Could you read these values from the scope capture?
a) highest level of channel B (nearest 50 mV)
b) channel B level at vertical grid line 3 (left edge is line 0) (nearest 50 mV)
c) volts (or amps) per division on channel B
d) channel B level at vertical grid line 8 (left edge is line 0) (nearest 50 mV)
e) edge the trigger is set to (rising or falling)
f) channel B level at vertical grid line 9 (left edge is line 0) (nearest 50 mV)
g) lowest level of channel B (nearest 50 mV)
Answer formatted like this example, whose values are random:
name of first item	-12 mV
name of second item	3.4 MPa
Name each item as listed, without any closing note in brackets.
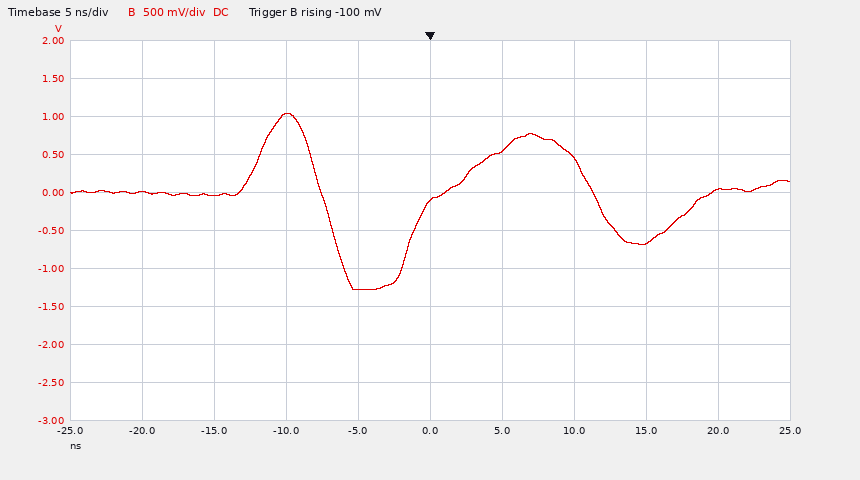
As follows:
highest level of channel B	1.05 V
channel B level at vertical grid line 3 (left edge is line 0)	1.05 V
volts (or amps) per division on channel B	500 mV
channel B level at vertical grid line 8 (left edge is line 0)	-650 mV
edge the trigger is set to	rising
channel B level at vertical grid line 9 (left edge is line 0)	50 mV
lowest level of channel B	-1.30 V
